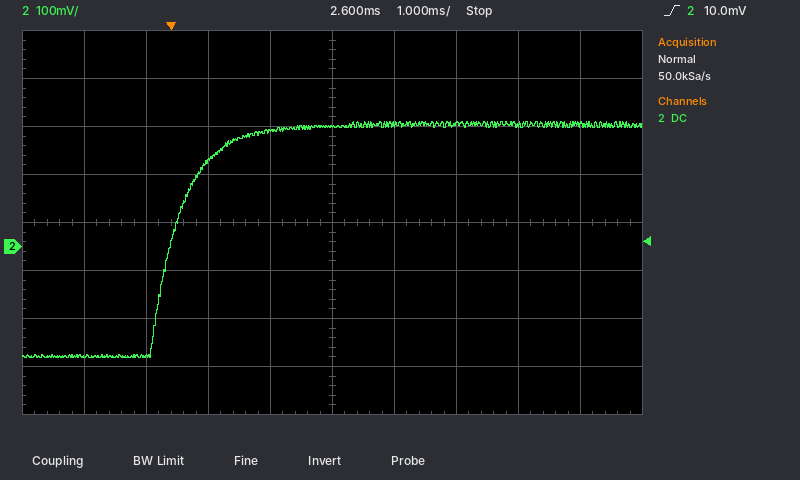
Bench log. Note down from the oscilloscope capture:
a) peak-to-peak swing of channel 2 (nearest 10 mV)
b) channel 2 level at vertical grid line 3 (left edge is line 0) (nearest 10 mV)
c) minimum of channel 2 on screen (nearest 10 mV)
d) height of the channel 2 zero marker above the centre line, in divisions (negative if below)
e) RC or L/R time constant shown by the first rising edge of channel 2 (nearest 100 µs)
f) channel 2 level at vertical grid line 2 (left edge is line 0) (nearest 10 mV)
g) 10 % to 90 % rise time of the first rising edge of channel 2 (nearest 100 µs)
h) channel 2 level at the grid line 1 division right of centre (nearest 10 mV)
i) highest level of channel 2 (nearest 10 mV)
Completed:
490 mV
180 mV
-230 mV
-0.5 div
500 µs
-230 mV
1.1 ms
250 mV
260 mV
